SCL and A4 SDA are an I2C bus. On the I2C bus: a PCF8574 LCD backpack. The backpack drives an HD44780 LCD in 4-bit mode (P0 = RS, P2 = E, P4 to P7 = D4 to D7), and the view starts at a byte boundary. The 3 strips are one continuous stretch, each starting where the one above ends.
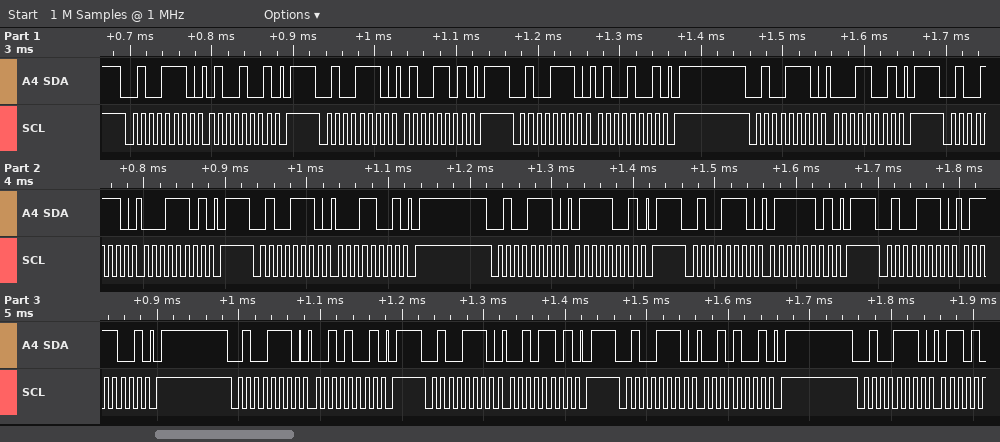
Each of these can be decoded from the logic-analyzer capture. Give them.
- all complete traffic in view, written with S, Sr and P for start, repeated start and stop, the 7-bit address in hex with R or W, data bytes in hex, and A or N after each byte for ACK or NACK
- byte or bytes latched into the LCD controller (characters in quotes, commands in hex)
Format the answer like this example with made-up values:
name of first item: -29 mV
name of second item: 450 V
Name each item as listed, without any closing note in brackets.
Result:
all complete traffic in view, written with S, Sr and P for start, repeated start and stop, the 7-bit address in hex with R or W, data bytes in hex, and A or N after each byte for ACK or NACK: S 27W A 49 A P S 27W A 4D A P S 27W A 49 A P S 27W A 19 A P S 27W A 1D A P S 27W A 19 A P S 27W A 79 A P S 27W A 7D A P S 27W A 79 A P S 27W A 29 A P S 27W A 2D A P S 27W A 29 A P S 27W A
byte or bytes latched into the LCD controller: 'A' 'r'
